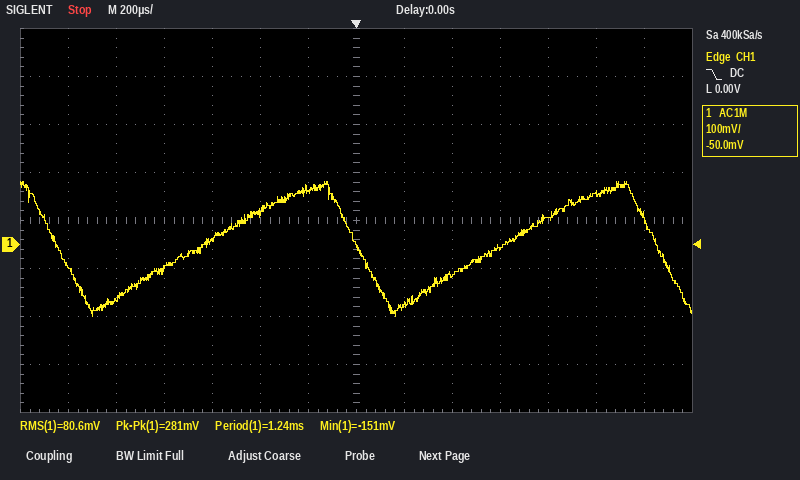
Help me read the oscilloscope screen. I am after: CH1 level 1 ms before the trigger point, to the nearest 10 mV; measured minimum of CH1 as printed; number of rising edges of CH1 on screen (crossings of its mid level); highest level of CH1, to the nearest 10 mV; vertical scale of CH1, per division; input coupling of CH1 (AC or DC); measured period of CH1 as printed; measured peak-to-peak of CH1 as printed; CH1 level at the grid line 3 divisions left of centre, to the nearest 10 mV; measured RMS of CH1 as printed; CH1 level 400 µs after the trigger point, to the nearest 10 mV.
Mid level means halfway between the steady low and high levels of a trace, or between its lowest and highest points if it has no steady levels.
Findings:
-110 mV
-151 mV
2
130 mV
100 mV
AC
1.24 ms
281 mV
10 mV
80.6 mV
-70 mV
